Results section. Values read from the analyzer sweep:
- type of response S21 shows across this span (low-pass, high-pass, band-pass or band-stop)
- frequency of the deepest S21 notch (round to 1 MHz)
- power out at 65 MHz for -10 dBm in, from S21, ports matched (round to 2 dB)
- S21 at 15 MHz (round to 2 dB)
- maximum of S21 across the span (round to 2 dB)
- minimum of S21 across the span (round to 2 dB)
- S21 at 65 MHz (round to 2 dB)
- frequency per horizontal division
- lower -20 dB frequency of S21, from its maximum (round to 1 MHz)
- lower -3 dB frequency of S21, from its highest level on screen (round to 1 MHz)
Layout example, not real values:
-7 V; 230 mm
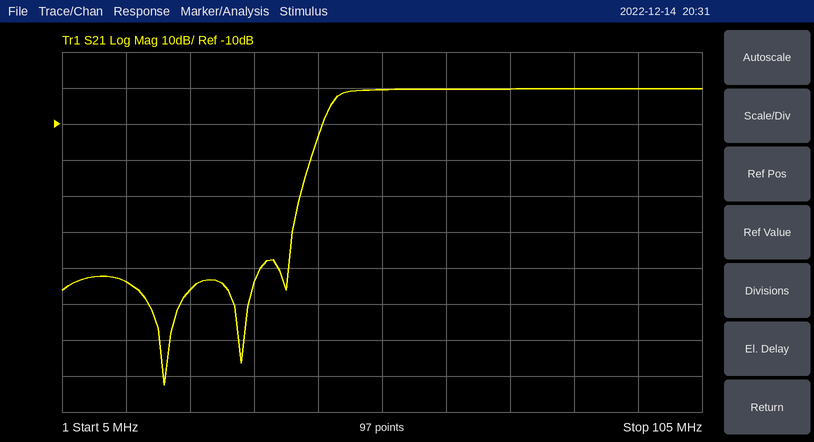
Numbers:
high-pass; 21 MHz; -10 dBm; -54 dB; 0 dB; -82 dB; 0 dB; 10 MHz; 44 MHz; 48 MHz
